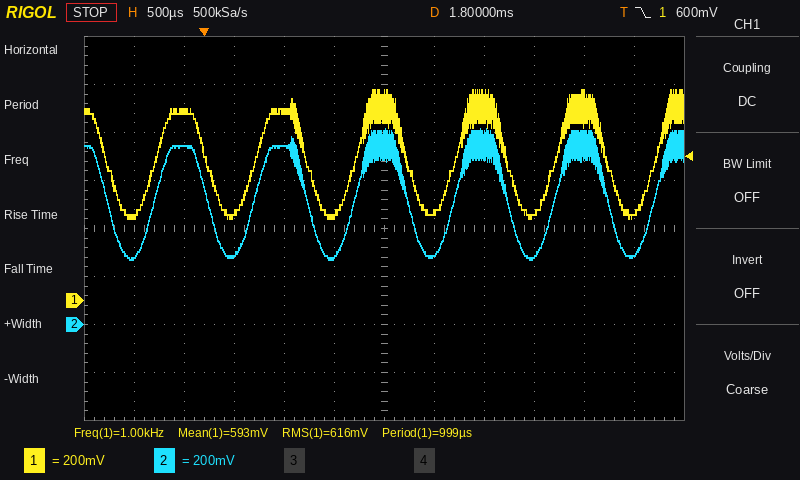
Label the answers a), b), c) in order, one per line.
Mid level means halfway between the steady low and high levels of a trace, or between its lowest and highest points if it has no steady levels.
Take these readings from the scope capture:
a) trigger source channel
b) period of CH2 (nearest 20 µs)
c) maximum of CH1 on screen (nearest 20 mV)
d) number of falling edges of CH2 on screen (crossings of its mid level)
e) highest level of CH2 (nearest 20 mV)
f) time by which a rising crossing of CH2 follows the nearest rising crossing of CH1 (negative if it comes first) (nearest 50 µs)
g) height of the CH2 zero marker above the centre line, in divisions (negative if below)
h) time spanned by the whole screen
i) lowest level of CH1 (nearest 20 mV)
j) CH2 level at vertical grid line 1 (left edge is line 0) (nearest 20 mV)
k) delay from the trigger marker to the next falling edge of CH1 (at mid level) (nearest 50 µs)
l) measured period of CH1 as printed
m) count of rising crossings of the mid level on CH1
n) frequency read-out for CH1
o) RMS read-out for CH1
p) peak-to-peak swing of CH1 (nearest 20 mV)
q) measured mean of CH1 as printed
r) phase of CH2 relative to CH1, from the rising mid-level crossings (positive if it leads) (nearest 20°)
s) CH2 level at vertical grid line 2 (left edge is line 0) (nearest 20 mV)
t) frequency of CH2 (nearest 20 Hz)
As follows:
a) CH1
b) 1.00 ms
c) 880 mV
d) 6
e) 820 mV
f) 0 µs
g) -2.0 div
h) 6 ms
i) 340 mV
j) 280 mV
k) 1.00 ms
l) 999 µs
m) 6
n) 1.00 kHz
o) 616 mV
p) 540 mV
q) 593 mV
r) 0°
s) 740 mV
t) 1.00 kHz
